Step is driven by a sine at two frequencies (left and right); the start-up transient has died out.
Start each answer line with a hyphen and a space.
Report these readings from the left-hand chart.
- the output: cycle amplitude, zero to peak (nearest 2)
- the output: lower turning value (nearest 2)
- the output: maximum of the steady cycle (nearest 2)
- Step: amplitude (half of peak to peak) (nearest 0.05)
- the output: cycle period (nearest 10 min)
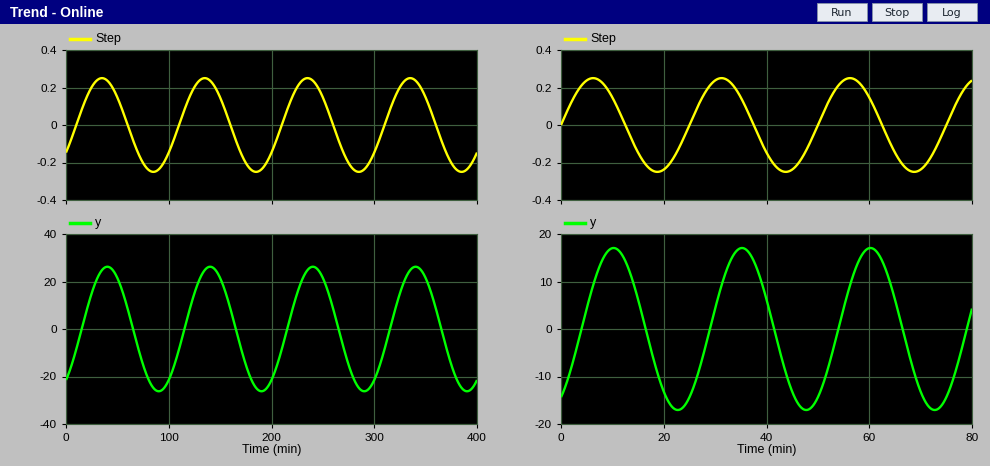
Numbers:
- 26
- -26
- 26
- 0.25
- 100 min
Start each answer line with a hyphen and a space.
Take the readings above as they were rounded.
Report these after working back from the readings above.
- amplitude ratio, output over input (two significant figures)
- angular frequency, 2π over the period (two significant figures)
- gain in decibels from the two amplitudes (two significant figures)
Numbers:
- 100
- 0.063 rad/min
- 40 dB
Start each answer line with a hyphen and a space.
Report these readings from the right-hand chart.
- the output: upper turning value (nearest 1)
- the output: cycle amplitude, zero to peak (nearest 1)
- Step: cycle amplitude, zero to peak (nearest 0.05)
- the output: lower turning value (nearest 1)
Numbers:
- 17
- 17
- 0.25
- -17
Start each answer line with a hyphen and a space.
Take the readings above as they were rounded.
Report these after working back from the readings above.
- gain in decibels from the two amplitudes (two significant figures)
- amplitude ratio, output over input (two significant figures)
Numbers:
- 37 dB
- 68
